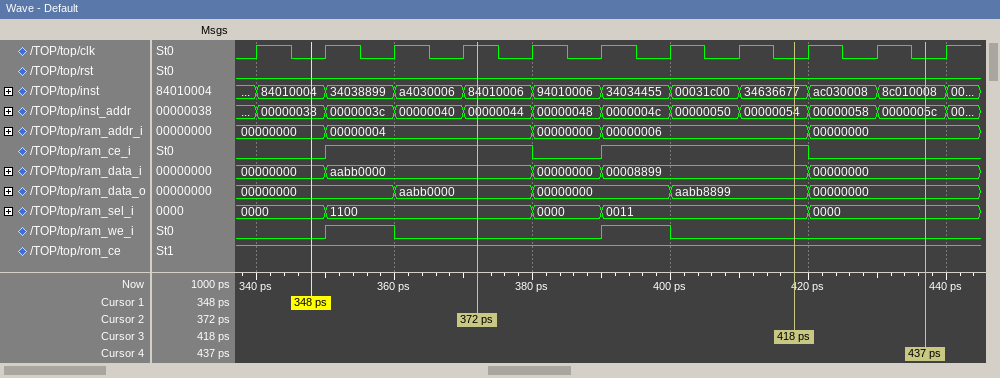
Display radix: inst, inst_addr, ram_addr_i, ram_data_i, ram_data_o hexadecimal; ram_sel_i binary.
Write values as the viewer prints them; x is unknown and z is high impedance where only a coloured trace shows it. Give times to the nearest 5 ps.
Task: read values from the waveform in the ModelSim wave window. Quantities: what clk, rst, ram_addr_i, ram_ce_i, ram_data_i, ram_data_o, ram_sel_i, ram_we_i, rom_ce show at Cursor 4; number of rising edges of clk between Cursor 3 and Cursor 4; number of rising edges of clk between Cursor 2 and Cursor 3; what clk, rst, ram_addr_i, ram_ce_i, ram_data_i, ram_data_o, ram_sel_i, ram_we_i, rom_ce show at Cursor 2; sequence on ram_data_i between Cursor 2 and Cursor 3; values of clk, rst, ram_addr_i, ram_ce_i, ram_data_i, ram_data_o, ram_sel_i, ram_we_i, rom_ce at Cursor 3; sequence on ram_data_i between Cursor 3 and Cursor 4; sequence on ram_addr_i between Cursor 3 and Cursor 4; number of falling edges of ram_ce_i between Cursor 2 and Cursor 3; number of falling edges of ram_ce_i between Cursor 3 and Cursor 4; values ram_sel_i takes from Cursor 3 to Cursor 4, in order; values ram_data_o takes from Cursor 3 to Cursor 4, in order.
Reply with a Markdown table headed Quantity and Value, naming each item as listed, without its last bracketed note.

| Quantity | Value |
|---|---|
| what clk, rst, ram_addr_i, ram_ce_i, ram_data_i, ram_data_o, ram_sel_i, ram_we_i, rom_ce show at Cursor 4 | clk=0, rst=0, ram_addr_i=00000000, ram_ce_i=0, ram_data_i=00000000, ram_data_o=00000000, ram_sel_i=0000, ram_we_i=0, rom_ce=1 |
| number of rising edges of clk between Cursor 3 and Cursor 4 | 2 |
| number of rising edges of clk between Cursor 2 and Cursor 3 | 4 |
| what clk, rst, ram_addr_i, ram_ce_i, ram_data_i, ram_data_o, ram_sel_i, ram_we_i, rom_ce show at Cursor 2 | clk=1, rst=0, ram_addr_i=00000004, ram_ce_i=1, ram_data_i=aabb0000, ram_data_o=aabb0000, ram_sel_i=1100, ram_we_i=0, rom_ce=1 |
| sequence on ram_data_i between Cursor 2 and Cursor 3 | aabb0000, 00000000, 00008899 |
| values of clk, rst, ram_addr_i, ram_ce_i, ram_data_i, ram_data_o, ram_sel_i, ram_we_i, rom_ce at Cursor 3 | clk=0, rst=0, ram_addr_i=00000006, ram_ce_i=1, ram_data_i=00008899, ram_data_o=aabb8899, ram_sel_i=0011, ram_we_i=0, rom_ce=1 |
| sequence on ram_data_i between Cursor 3 and Cursor 4 | 00008899, 00000000 |
| sequence on ram_addr_i between Cursor 3 and Cursor 4 | 00000006, 00000000 |
| number of falling edges of ram_ce_i between Cursor 2 and Cursor 3 | 1 |
| number of falling edges of ram_ce_i between Cursor 3 and Cursor 4 | 1 |
| values ram_sel_i takes from Cursor 3 to Cursor 4, in order | 0011, 0000 |
| values ram_data_o takes from Cursor 3 to Cursor 4, in order | aabb8899, 00000000 |
